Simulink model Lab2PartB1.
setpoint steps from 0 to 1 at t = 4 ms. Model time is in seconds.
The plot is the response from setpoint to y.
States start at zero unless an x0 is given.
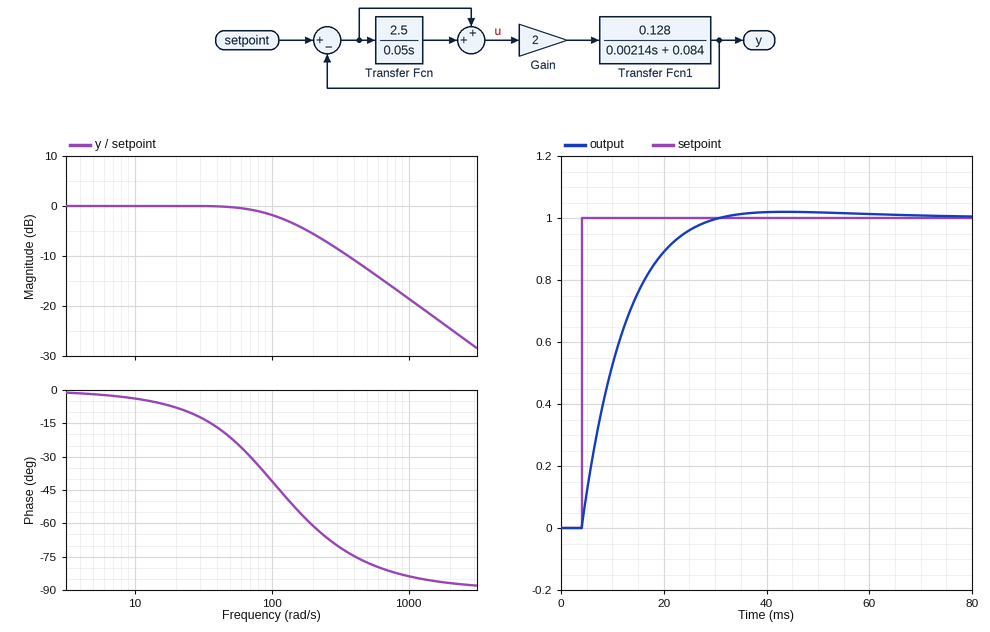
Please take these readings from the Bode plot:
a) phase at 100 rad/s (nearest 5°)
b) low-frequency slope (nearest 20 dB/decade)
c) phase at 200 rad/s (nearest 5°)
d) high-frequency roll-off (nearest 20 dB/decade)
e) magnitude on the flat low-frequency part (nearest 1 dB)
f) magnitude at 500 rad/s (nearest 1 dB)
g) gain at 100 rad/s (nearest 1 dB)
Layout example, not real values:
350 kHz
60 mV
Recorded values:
-40°
0 dB/decade
-60°
-20 dB/decade
0 dB
-13 dB
-2 dB
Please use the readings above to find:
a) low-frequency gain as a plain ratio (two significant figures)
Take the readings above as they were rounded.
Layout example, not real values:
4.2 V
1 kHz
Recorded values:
1.0
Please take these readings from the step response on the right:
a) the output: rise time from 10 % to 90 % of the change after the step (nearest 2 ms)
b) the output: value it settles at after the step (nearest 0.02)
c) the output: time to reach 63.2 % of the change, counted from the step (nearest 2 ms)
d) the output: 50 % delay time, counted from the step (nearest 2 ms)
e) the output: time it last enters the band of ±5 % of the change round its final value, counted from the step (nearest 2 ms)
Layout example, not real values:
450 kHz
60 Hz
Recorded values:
16 ms
1.00
8 ms
6 ms
20 ms
